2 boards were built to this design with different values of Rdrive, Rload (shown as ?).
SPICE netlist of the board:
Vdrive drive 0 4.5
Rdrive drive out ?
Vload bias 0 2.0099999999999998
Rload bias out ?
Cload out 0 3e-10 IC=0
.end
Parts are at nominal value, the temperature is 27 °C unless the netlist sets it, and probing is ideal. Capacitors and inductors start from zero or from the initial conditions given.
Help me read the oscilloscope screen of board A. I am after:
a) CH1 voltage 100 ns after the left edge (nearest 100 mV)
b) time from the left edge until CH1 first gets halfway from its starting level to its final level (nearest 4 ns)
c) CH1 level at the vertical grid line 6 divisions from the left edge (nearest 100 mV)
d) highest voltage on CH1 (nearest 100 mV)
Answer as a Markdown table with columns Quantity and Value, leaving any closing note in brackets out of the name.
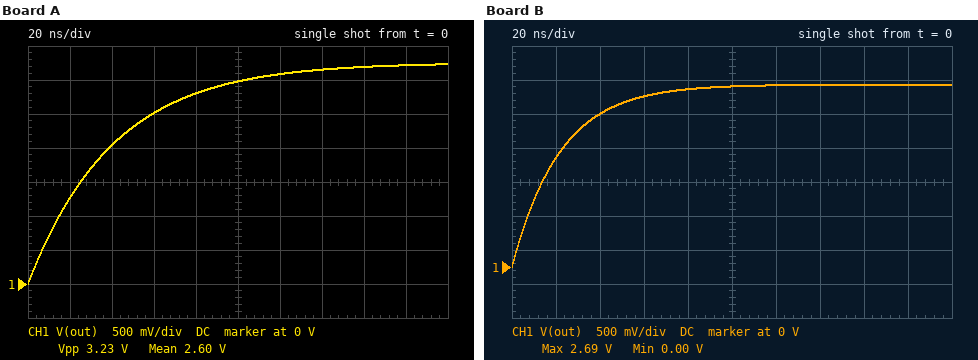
| Quantity | Value |
|---|---|
| CH1 voltage 100 ns after the left edge | 3.0 V |
| time from the left edge until CH1 first gets halfway from its starting level to its final level | 28 ns |
| CH1 level at the vertical grid line 6 divisions from the left edge | 3.1 V |
| highest voltage on CH1 | 3.2 V |
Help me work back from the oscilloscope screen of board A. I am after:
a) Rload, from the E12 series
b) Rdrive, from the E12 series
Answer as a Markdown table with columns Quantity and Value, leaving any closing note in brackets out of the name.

| Quantity | Value |
|---|---|
| Rload, from the E12 series | 270 Ω |
| Rdrive, from the E12 series | 270 Ω |
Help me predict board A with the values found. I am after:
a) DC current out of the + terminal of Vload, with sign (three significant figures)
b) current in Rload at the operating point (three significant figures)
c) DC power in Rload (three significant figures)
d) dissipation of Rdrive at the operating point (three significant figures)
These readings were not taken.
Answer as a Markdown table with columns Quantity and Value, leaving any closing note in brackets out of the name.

| Quantity | Value |
|---|---|
| DC current out of the + terminal of Vload, with sign | -4.61 mA |
| current in Rload at the operating point | 4.61 mA |
| DC power in Rload | 5.74 mW |
| dissipation of Rdrive at the operating point | 5.74 mW |
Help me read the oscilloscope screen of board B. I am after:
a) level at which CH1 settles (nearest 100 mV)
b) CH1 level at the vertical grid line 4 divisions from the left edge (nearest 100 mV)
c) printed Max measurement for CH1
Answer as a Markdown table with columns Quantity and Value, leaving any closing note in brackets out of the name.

| Quantity | Value |
|---|---|
| level at which CH1 settles | 2.7 V |
| CH1 level at the vertical grid line 4 divisions from the left edge | 2.6 V |
| printed Max measurement for CH1 | 2.69 V |
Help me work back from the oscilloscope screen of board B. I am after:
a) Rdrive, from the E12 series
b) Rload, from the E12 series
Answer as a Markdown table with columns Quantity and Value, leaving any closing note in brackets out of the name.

| Quantity | Value |
|---|---|
| Rdrive, from the E12 series | 270 Ω |
| Rload, from the E12 series | 100 Ω |
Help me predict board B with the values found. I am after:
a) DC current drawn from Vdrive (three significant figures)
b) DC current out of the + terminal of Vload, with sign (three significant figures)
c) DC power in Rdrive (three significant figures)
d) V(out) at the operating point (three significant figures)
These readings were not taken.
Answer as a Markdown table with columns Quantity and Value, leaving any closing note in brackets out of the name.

| Quantity | Value |
|---|---|
| DC current drawn from Vdrive | 6.73 mA |
| DC current out of the + terminal of Vload, with sign | -6.73 mA |
| DC power in Rdrive | 12.2 mW |
| V(out) at the operating point | 2.68 V |
